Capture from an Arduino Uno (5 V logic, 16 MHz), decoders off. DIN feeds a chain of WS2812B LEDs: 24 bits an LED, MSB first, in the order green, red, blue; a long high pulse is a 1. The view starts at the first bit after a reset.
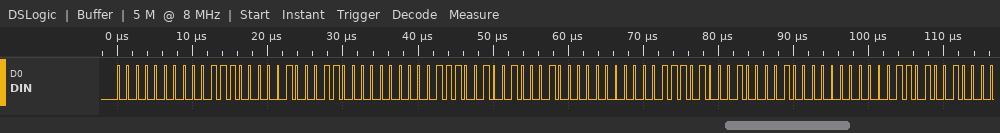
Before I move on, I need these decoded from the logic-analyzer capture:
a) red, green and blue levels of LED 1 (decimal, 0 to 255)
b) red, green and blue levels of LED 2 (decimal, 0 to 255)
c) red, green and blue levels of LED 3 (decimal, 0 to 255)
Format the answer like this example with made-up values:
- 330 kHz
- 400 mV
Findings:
- 56, 0, 35
- 57, 0, 34
- 58, 0, 33
